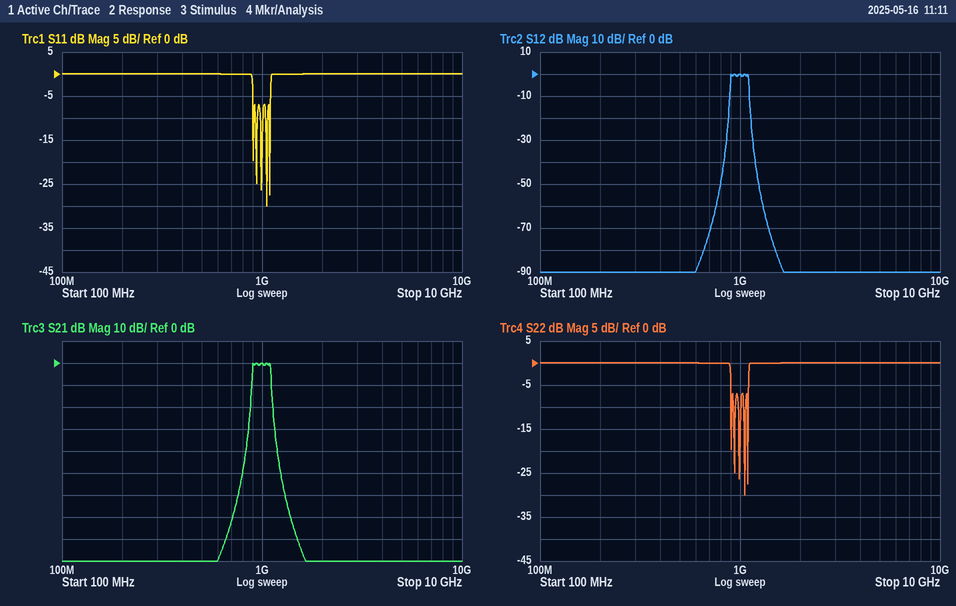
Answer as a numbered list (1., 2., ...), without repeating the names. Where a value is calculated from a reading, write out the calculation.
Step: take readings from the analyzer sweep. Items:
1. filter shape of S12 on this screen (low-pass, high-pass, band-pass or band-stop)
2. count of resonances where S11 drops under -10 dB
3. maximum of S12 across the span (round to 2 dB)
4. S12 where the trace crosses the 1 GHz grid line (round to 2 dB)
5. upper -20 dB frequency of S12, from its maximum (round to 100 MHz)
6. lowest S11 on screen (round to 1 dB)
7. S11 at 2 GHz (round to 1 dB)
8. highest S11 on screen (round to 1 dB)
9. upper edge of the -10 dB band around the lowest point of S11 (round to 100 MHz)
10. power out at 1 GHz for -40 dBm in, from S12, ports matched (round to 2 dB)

1. band-pass
2. 5
3. 0 dB
4. 0 dB
5. 1.1 GHz
6. -30 dB
7. 0 dB
8. 0 dB
9. 1.1 GHz
10. -40 dBm + (0 dB) = -40 dBm
